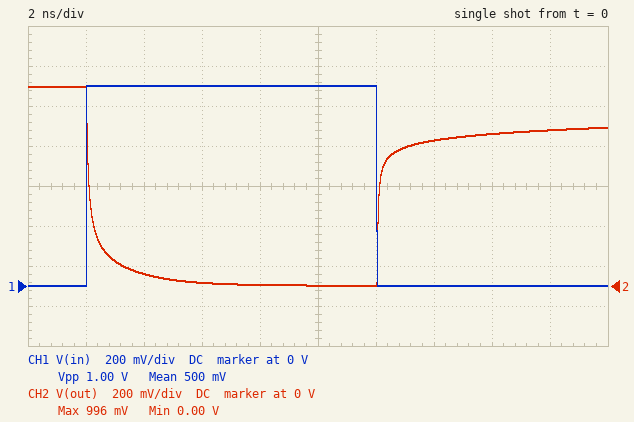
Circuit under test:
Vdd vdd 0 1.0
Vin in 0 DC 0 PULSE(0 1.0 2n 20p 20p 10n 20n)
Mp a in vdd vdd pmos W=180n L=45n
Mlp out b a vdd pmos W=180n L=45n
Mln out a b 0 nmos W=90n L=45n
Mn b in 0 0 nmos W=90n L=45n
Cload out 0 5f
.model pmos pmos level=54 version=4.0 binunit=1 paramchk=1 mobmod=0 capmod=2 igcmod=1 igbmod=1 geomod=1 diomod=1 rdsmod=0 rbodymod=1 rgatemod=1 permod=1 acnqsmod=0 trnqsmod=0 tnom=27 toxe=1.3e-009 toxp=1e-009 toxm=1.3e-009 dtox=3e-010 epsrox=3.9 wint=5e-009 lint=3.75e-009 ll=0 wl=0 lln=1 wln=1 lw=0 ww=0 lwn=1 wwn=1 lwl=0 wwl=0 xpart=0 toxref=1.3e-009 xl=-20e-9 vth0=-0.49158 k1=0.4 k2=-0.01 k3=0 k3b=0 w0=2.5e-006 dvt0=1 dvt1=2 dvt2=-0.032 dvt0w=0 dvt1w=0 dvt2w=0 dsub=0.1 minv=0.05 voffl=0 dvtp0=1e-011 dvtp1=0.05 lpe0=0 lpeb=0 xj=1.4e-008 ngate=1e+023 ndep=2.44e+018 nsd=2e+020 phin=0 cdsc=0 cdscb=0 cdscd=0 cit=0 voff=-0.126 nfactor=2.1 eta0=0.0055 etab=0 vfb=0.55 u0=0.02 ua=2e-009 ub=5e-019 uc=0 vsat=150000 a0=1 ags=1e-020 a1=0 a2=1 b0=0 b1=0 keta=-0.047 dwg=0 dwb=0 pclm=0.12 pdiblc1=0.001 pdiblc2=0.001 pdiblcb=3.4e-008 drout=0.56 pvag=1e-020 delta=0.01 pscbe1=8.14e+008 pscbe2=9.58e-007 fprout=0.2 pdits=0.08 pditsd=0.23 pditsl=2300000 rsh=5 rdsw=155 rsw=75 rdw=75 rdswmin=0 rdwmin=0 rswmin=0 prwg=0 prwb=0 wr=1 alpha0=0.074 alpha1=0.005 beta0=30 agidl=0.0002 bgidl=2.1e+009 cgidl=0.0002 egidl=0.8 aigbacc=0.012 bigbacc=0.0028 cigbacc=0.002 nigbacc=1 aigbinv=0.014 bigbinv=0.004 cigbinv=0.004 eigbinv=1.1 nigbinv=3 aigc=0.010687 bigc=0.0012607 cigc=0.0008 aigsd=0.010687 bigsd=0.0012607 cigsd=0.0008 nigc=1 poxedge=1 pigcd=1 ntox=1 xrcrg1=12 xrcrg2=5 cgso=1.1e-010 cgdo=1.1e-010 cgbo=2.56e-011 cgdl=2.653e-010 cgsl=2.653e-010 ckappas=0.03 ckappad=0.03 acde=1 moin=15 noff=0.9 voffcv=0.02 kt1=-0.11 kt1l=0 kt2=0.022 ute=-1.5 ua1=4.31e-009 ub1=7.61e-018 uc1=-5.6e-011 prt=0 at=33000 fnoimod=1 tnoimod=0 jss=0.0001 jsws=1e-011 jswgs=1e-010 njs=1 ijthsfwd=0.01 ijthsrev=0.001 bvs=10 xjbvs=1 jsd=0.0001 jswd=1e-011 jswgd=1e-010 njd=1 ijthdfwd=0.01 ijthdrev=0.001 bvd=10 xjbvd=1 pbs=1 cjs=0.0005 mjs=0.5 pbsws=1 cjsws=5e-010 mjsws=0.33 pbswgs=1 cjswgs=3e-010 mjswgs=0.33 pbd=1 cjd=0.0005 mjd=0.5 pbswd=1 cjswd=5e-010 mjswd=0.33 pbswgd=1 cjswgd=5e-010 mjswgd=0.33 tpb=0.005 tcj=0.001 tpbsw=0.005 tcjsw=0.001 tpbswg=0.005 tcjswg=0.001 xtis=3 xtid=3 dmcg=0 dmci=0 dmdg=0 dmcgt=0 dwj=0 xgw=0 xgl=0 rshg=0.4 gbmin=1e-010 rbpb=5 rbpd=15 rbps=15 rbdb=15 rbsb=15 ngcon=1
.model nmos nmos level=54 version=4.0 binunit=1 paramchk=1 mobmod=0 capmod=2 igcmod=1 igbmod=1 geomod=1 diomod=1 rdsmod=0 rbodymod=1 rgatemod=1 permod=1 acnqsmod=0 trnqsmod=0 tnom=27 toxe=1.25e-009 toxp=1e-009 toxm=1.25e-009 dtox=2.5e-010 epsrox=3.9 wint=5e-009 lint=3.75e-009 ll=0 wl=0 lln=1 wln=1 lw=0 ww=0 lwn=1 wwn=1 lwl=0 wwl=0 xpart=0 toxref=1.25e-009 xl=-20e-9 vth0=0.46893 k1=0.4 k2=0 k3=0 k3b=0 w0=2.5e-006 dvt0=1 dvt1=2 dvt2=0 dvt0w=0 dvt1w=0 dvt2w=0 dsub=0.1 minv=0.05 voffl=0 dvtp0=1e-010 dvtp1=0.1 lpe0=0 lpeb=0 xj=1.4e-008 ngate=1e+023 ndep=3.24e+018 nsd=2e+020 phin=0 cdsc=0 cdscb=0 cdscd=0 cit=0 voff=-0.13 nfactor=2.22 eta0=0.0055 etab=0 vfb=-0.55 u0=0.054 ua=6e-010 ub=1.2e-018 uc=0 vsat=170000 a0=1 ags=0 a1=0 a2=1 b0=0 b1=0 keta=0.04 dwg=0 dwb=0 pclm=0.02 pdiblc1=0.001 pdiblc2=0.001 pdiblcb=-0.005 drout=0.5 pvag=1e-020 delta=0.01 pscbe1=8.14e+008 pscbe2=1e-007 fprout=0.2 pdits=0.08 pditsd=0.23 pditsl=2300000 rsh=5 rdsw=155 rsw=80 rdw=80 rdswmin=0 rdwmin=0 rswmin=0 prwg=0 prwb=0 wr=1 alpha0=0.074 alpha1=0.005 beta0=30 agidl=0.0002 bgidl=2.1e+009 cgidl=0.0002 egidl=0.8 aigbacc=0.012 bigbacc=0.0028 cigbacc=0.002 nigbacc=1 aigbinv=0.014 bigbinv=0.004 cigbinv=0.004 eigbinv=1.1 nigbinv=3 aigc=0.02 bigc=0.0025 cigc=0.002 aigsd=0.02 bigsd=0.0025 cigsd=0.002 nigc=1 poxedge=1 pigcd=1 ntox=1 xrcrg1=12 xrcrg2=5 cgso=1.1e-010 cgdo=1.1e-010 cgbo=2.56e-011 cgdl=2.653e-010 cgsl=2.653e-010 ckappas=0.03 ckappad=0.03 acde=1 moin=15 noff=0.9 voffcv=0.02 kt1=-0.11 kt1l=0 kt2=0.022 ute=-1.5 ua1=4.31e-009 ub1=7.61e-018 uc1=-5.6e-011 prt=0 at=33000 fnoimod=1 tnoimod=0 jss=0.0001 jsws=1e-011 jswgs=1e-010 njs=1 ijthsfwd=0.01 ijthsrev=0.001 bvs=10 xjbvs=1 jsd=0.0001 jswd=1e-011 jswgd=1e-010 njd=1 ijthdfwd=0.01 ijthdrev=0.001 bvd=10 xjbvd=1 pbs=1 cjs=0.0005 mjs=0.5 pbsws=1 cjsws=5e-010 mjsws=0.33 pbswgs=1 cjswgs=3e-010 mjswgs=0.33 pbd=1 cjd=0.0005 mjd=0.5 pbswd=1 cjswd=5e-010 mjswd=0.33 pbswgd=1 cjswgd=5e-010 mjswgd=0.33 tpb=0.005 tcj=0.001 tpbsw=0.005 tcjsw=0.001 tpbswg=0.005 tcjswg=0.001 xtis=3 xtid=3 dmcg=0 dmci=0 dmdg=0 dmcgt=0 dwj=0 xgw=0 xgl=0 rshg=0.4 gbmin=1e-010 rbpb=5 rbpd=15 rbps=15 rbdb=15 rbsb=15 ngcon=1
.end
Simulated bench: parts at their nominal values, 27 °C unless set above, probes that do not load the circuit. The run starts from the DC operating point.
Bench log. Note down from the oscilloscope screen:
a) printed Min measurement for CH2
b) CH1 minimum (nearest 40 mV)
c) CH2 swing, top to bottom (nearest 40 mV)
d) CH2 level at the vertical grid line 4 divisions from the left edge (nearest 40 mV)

0.00 V
0 V
1.00 V
0 V
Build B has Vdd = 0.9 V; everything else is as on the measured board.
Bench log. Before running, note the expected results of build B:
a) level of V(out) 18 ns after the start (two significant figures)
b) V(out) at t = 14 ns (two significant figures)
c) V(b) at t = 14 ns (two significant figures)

660 mV
610 mV
590 mV
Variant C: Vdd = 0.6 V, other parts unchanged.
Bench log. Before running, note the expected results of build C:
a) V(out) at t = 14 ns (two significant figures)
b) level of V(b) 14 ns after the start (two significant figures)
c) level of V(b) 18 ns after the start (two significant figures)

300 mV
290 mV
330 mV
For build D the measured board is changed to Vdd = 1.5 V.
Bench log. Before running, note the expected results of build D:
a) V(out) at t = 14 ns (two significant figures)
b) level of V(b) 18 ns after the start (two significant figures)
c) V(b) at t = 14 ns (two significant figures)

1.4 V
1.2 V
1.1 V
